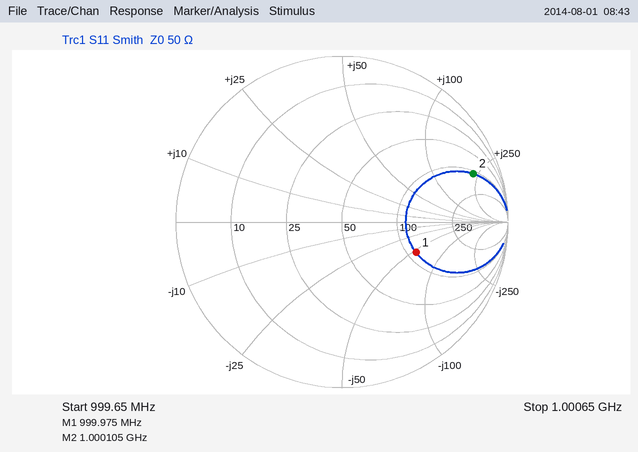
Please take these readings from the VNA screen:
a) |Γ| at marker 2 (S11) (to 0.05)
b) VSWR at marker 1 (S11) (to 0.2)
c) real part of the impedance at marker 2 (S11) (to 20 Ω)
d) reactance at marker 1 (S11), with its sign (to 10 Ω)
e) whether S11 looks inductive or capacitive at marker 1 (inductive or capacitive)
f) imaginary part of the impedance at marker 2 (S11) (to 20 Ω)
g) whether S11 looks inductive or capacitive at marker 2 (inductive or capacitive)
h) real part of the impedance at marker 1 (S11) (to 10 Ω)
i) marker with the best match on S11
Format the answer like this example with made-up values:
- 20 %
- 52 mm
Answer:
- 0.85
- 2.8
- 120 Ω
- -50 Ω
- capacitive
- +220 Ω
- inductive
- 110 Ω
- marker 1
